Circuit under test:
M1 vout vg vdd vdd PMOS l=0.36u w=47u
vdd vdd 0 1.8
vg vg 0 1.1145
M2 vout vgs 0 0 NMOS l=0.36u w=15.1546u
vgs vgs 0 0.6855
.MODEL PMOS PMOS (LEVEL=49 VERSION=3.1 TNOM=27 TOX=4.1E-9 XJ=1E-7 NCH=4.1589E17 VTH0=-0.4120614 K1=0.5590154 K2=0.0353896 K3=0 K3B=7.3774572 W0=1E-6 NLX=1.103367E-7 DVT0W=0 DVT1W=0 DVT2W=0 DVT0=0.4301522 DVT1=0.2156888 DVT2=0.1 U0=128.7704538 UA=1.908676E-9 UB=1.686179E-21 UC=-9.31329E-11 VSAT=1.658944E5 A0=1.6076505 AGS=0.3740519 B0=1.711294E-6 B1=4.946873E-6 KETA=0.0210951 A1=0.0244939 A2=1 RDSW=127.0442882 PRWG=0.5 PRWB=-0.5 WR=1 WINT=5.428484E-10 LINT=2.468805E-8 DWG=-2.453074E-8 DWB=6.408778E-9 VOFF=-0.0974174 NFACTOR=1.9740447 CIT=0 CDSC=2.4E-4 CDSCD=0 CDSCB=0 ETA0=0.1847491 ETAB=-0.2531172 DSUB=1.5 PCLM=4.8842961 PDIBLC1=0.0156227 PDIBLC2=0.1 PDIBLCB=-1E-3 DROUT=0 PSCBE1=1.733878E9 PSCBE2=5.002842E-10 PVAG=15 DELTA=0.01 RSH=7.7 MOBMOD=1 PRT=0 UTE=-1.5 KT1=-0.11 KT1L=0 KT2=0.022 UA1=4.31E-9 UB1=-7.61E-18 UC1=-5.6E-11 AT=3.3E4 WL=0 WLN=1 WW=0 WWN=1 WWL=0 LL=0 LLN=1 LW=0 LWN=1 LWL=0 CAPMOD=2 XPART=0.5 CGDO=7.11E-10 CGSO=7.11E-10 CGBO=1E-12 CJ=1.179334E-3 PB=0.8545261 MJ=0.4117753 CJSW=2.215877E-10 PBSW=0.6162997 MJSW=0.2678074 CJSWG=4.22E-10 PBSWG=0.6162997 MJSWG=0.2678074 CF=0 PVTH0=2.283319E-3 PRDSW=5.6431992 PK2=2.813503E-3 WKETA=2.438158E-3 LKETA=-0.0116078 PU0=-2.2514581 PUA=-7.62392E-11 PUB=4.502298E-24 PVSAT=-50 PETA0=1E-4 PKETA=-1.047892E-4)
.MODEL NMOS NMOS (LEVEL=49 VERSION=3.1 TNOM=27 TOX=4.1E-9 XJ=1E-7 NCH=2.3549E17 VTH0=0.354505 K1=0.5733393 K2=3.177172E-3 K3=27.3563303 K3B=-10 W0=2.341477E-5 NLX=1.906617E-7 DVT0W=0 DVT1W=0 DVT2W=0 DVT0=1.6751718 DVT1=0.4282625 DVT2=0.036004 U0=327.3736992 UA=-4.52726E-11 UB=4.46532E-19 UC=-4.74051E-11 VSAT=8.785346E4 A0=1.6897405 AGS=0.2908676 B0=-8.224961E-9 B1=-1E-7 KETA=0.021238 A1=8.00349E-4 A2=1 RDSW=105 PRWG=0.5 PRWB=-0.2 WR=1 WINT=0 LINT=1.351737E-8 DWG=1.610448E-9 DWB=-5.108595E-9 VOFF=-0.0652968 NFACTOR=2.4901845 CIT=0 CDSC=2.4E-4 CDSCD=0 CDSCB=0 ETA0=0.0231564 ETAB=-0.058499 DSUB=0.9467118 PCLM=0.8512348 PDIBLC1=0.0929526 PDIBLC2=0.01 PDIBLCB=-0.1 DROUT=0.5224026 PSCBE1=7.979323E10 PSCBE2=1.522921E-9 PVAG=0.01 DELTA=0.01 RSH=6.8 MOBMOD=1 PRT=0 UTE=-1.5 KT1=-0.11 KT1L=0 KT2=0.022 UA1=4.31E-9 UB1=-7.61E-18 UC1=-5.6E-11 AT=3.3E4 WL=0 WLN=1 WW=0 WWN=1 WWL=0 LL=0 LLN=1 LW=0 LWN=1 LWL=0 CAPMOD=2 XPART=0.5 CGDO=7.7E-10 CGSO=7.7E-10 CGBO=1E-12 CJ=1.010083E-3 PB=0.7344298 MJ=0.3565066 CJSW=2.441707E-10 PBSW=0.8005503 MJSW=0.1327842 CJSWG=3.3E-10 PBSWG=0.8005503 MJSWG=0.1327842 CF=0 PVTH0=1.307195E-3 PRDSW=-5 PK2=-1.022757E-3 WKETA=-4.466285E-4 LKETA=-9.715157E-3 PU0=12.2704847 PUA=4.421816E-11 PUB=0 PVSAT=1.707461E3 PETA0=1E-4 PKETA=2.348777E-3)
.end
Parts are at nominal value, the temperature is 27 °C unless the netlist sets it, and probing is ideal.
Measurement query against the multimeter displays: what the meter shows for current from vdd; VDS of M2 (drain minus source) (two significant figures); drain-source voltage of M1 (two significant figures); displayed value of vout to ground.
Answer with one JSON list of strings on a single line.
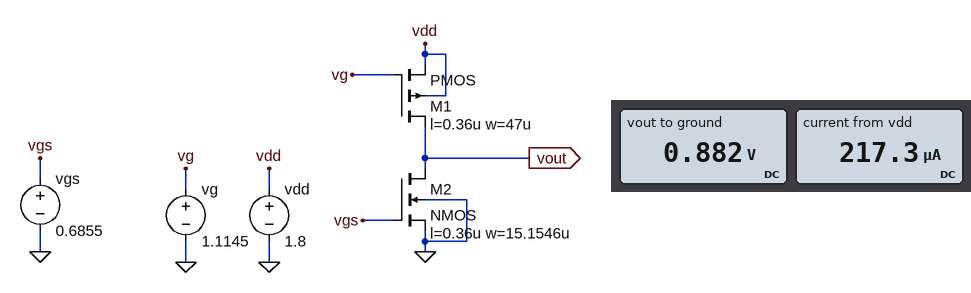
["217.3 µA", "880 mV", "-920 mV", "0.882 V"]
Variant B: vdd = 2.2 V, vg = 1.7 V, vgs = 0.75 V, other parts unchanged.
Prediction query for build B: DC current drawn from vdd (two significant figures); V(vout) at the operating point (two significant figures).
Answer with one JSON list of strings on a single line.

["19 µA", "6.4 mV"]
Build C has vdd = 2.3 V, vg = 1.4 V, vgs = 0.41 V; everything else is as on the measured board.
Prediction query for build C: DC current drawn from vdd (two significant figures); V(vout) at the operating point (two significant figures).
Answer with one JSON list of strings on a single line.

["1.8 µA", "2.3 V"]
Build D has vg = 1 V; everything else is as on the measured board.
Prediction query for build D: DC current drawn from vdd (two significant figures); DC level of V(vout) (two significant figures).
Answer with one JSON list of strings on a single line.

["230 µA", "1.7 V"]
